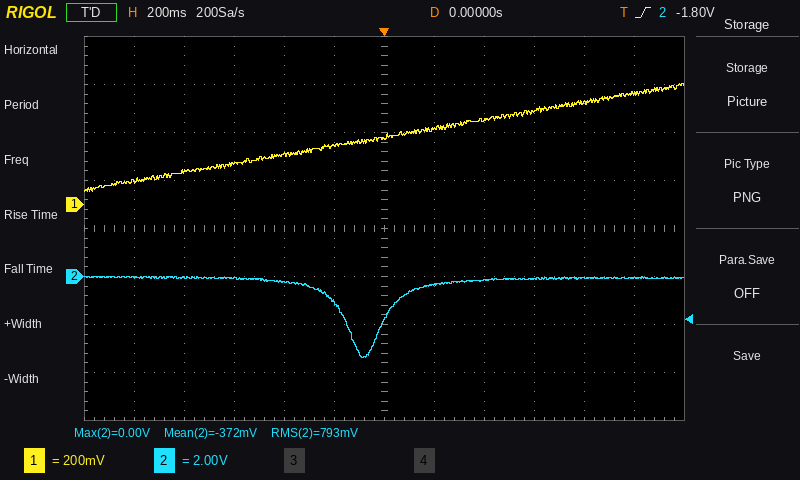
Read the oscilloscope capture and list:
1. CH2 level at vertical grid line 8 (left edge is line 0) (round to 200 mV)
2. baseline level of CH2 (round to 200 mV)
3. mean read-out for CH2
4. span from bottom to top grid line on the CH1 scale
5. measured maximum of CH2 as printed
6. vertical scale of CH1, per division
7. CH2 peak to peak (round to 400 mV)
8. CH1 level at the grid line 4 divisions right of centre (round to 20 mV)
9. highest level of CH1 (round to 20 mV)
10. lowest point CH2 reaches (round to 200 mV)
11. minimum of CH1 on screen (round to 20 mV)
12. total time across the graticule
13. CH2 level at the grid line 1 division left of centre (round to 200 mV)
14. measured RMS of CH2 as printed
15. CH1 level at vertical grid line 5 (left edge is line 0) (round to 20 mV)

-200 mV
0.0 V
-372 mV
1.6 V
0.00 V
200 mV
3.2 V
420 mV
500 mV
-3.4 V
60 mV
2.4 s
-1.0 V
793 mV
240 mV
